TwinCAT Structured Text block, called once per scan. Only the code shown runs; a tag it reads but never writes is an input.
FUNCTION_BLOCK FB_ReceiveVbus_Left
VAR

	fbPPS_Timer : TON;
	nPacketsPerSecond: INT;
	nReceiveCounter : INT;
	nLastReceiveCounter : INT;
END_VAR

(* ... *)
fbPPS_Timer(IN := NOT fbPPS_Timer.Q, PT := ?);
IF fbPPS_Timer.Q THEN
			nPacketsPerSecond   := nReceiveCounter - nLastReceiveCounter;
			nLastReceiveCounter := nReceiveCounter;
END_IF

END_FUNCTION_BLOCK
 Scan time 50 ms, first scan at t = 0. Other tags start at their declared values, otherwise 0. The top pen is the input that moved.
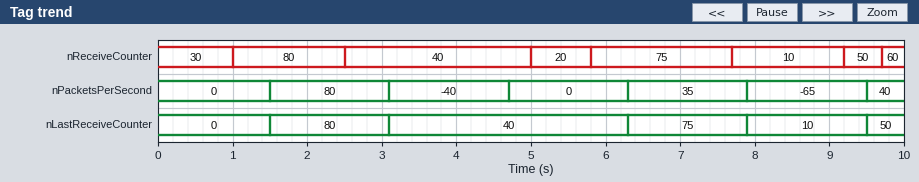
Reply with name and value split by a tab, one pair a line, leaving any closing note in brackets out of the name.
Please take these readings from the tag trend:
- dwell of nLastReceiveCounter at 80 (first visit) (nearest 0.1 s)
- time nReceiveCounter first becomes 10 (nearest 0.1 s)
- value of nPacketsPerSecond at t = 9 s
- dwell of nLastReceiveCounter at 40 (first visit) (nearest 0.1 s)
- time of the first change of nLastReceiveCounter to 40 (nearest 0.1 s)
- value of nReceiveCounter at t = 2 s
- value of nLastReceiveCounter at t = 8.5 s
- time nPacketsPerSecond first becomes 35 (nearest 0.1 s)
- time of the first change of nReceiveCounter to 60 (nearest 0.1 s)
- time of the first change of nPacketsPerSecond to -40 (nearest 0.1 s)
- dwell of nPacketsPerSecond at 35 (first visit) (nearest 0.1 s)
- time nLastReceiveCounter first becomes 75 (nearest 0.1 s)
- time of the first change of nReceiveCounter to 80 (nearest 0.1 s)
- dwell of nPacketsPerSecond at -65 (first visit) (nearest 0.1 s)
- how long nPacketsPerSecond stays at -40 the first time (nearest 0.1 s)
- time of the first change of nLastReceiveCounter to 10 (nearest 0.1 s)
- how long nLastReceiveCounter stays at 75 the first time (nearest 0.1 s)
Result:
dwell of nLastReceiveCounter at 80 (first visit)	1.6 s
time nReceiveCounter first becomes 10	7.7 s
value of nPacketsPerSecond at t = 9 s	-65
dwell of nLastReceiveCounter at 40 (first visit)	3.2 s
time of the first change of nLastReceiveCounter to 40	3.1 s
value of nReceiveCounter at t = 2 s	80
value of nLastReceiveCounter at t = 8.5 s	10
time nPacketsPerSecond first becomes 35	6.3 s
time of the first change of nReceiveCounter to 60	9.7 s
time of the first change of nPacketsPerSecond to -40	3.1 s
dwell of nPacketsPerSecond at 35 (first visit)	1.6 s
time nLastReceiveCounter first becomes 75	6.3 s
time of the first change of nReceiveCounter to 80	1.0 s
dwell of nPacketsPerSecond at -65 (first visit)	1.6 s
how long nPacketsPerSecond stays at -40 the first time	1.6 s
time of the first change of nLastReceiveCounter to 10	7.9 s
how long nLastReceiveCounter stays at 75 the first time	1.6 s
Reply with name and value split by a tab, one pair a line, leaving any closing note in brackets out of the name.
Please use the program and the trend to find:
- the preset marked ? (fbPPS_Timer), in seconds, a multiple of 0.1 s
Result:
the preset marked ? (fbPPS_Timer), in seconds, a multiple of 0.1 s	1.5 s
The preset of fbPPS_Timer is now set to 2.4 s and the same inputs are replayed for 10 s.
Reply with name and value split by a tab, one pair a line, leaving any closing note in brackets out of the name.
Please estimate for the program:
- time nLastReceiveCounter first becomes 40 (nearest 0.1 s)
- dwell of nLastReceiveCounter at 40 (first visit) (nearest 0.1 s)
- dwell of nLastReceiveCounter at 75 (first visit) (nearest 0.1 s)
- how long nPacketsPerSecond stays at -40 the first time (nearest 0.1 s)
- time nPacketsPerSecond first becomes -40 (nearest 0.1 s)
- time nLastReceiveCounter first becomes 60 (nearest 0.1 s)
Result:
time nLastReceiveCounter first becomes 40	4.9 s
dwell of nLastReceiveCounter at 40 (first visit)	2.5 s
dwell of nLastReceiveCounter at 75 (first visit)	2.5 s
how long nPacketsPerSecond stays at -40 the first time	2.5 s
time nPacketsPerSecond first becomes -40	4.9 s
time nLastReceiveCounter first becomes 60	9.9 s
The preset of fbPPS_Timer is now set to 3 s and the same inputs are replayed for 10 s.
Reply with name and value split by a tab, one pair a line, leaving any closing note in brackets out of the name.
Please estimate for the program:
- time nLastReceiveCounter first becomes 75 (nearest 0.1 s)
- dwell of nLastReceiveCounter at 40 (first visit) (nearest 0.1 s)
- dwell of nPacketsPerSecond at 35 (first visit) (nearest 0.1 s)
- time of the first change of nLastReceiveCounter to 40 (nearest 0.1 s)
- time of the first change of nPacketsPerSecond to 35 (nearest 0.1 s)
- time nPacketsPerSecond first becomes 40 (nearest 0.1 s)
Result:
time nLastReceiveCounter first becomes 75	6.1 s
dwell of nLastReceiveCounter at 40 (first visit)	3.1 s
dwell of nPacketsPerSecond at 35 (first visit)	3.1 s
time of the first change of nLastReceiveCounter to 40	3.0 s
time of the first change of nPacketsPerSecond to 35	6.1 s
time nPacketsPerSecond first becomes 40	3.0 s
